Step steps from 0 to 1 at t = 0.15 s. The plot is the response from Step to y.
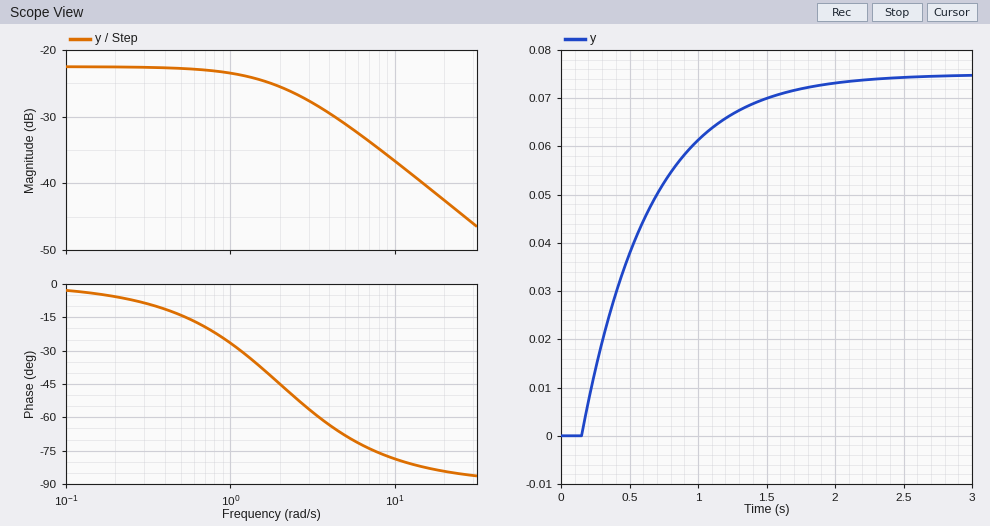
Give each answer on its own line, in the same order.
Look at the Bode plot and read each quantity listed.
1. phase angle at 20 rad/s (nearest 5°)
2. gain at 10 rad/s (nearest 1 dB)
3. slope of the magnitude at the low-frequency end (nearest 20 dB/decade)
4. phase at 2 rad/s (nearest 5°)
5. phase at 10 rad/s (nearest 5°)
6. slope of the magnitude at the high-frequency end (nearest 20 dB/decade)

-85°
-37 dB
0 dB/decade
-45°
-80°
-20 dB/decade
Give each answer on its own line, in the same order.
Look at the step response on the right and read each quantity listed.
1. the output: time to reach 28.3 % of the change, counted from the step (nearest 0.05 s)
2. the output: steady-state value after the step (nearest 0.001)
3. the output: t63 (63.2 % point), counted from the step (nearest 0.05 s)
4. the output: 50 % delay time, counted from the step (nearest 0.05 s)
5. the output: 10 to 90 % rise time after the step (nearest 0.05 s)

0.15 s
0.075
0.50 s
0.35 s
1.10 s
